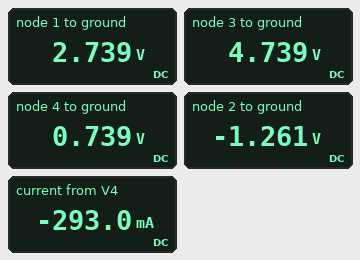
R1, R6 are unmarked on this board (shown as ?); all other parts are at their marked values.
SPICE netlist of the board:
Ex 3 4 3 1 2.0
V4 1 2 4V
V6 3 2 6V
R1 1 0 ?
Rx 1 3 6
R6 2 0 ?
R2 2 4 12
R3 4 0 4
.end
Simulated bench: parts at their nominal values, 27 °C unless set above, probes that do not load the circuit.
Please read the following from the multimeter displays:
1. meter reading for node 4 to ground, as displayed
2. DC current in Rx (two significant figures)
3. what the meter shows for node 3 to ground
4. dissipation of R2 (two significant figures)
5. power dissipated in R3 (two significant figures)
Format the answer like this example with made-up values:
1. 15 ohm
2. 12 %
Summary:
1. 0.739 V
2. 330 mA
3. 4.739 V
4. 330 mW
5. 140 mW
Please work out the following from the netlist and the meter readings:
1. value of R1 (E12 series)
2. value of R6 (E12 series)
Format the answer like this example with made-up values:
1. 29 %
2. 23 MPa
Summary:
1. 68 Ω
2. 5.6 Ω
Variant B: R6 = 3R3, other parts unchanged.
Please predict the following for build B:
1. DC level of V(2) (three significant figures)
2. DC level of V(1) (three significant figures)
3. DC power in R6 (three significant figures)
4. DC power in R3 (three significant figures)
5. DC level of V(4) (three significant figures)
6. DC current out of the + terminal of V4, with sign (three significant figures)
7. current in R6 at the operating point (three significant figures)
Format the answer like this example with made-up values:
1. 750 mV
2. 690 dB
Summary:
1. -984 mV
2. 3.02 V
3. 294 mW
4. 258 mW
5. 1.02 V
6. -289 mA
7. 298 mA
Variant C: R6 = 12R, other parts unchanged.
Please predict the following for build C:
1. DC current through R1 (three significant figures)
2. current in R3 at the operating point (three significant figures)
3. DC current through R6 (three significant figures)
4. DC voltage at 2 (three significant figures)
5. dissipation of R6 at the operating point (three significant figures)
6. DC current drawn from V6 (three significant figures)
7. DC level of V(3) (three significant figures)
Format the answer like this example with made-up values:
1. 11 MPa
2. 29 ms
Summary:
1. 35.2 mA
2. 98.6 mA
3. 134 mA
4. -1.61 V
5. 215 mW
6. 599 mA
7. 4.39 V
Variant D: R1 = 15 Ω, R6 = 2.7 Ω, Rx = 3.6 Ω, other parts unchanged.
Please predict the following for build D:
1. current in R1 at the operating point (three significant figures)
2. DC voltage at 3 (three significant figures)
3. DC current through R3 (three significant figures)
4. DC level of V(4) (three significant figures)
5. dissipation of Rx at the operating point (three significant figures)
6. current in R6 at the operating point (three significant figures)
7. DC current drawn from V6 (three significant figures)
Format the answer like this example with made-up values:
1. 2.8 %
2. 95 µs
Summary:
1. 192 mA
2. 4.88 V
3. 221 mA
4. 884 mV
5. 1.11 W
6. 413 mA
7. 943 mA
